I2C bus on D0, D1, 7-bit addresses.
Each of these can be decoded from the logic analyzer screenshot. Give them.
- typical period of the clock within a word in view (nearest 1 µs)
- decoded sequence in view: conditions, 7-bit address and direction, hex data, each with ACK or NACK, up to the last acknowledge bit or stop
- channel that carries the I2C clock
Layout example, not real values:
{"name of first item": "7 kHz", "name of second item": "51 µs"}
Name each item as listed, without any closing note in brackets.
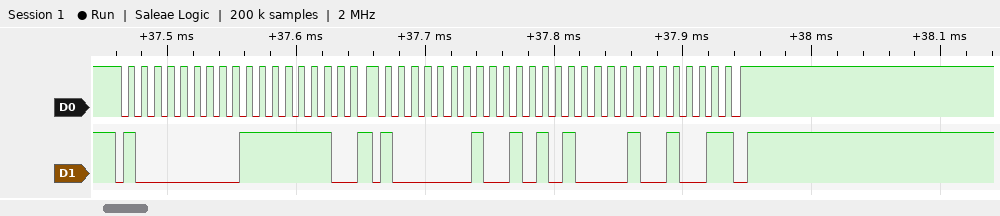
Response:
{"typical period of the clock within a word in view": "10 µs", "decoded sequence in view: conditions, 7-bit address and direction, hex data, each with ACK or NACK, up to the last acknowledge bit or stop": "start, address 40 write ACK, FE ACK, repeated start, address 40 read ACK, 54 ACK, 49 NACK, stop", "channel that carries the I2C clock": "D0"}
